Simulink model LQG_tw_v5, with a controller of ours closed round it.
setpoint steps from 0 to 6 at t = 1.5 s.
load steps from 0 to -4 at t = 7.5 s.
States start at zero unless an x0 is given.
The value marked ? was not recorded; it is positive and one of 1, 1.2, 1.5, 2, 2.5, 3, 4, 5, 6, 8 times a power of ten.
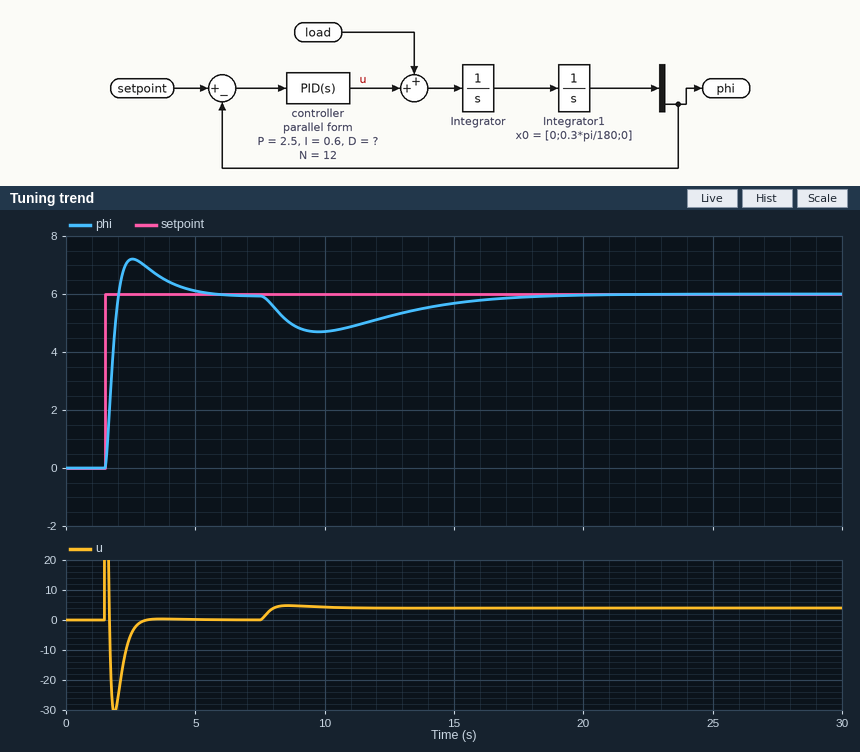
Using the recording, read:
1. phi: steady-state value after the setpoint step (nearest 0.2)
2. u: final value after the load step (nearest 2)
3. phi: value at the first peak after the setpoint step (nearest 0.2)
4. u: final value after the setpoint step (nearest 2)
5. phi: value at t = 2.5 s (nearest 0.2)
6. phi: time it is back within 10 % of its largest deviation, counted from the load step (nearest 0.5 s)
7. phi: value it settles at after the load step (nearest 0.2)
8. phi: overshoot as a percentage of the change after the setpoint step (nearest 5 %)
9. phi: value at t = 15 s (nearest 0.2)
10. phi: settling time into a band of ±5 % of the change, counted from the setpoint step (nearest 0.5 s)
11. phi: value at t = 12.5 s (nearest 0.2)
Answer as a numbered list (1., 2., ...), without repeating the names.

1. 6.0
2. 4
3. 7.2
4. 0
5. 7.2
6. 10.0 s
7. 6.0
8. 20 %
9. 5.6
10. 3.0 s
11. 5.2
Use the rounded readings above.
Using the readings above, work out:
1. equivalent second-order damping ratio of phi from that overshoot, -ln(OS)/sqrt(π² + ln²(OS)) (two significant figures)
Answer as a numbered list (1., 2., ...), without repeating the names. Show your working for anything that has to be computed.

1. ln(0.2) = -1.609; 1.609 / sqrt(9.870 + 2.590) = 0.46
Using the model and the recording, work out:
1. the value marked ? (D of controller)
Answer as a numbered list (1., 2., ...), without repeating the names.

1. 3
